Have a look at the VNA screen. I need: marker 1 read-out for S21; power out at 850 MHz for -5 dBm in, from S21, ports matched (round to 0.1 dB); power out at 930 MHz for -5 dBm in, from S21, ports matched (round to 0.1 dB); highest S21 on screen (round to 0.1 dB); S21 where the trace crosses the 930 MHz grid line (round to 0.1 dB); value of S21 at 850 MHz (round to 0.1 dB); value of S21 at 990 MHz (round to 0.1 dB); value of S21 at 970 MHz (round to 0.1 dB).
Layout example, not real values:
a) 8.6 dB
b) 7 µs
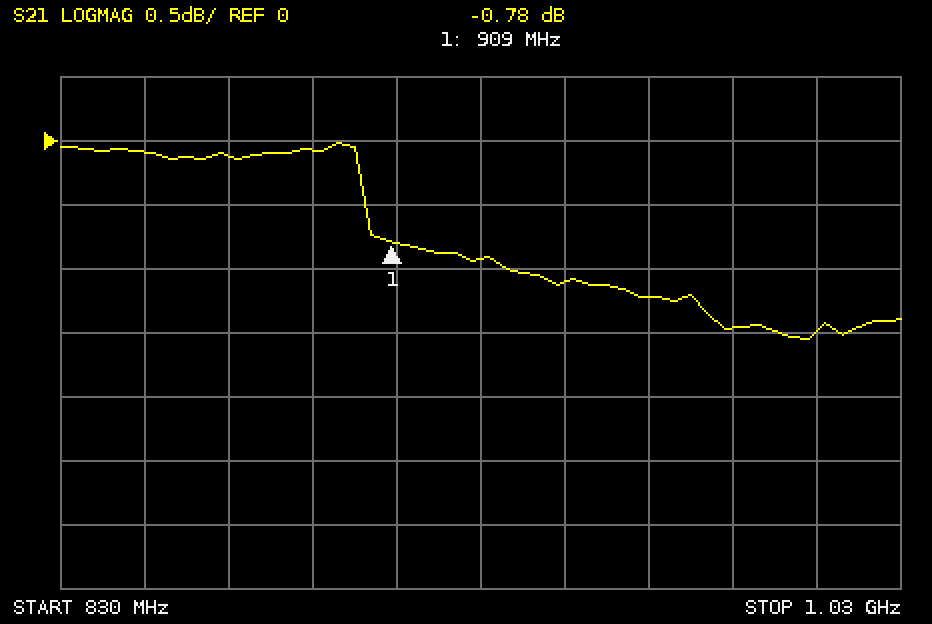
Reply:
a) -0.78 dB
b) -5.1 dBm
c) -5.9 dBm
d) 0.0 dB
e) -0.9 dB
f) -0.1 dB
g) -1.5 dB
h) -1.2 dB
